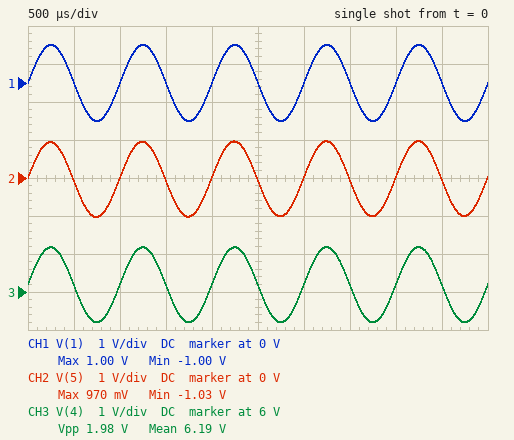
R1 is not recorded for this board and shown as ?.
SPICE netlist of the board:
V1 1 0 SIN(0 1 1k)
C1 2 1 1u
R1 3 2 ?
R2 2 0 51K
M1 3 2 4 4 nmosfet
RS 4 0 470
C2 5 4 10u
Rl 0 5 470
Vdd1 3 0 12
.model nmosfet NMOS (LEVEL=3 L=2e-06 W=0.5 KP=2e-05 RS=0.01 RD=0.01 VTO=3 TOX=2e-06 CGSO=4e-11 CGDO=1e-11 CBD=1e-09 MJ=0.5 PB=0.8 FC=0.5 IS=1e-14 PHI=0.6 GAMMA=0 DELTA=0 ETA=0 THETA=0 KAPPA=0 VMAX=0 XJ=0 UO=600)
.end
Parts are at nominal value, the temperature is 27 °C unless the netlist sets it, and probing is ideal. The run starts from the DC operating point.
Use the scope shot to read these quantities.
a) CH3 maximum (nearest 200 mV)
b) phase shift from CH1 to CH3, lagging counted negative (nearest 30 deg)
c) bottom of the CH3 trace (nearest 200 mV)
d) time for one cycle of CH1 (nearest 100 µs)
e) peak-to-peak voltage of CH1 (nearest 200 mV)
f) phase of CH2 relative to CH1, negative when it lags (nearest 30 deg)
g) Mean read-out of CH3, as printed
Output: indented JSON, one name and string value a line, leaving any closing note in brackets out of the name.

{
  "CH3 maximum": "7.2 V",
  "phase shift from CH1 to CH3, lagging counted negative": "0 deg",
  "bottom of the CH3 trace": "5.2 V",
  "time for one cycle of CH1": "1.0 ms",
  "peak-to-peak voltage of CH1": "2.0 V",
  "phase of CH2 relative to CH1, negative when it lags": "0 deg",
  "Mean read-out of CH3, as printed": "6.19 V"
}
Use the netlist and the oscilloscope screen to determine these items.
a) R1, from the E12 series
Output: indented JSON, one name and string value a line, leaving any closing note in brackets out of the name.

{
  "R1, from the E12 series": "15 kΩ"
}
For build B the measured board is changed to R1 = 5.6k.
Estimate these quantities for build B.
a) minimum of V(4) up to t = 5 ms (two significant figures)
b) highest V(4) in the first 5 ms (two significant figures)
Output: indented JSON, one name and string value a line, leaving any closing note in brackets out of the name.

{
  "minimum of V(4) up to t = 5 ms": "6.7 V",
  "highest V(4) in the first 5 ms": "8.7 V"
}
